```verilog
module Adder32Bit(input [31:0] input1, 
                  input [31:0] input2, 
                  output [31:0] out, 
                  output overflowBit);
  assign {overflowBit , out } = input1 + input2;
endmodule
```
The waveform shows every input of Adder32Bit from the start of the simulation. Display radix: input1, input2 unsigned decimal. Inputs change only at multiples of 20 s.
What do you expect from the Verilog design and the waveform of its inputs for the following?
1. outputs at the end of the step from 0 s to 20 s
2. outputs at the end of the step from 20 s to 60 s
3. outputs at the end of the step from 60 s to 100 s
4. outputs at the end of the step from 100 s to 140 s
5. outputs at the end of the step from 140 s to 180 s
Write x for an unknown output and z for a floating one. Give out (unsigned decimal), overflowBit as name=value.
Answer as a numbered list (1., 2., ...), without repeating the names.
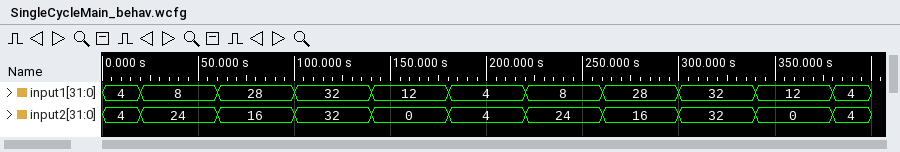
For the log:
1. out=8, overflowBit=0
2. out=32, overflowBit=0
3. out=44, overflowBit=0
4. out=64, overflowBit=0
5. out=12, overflowBit=0
